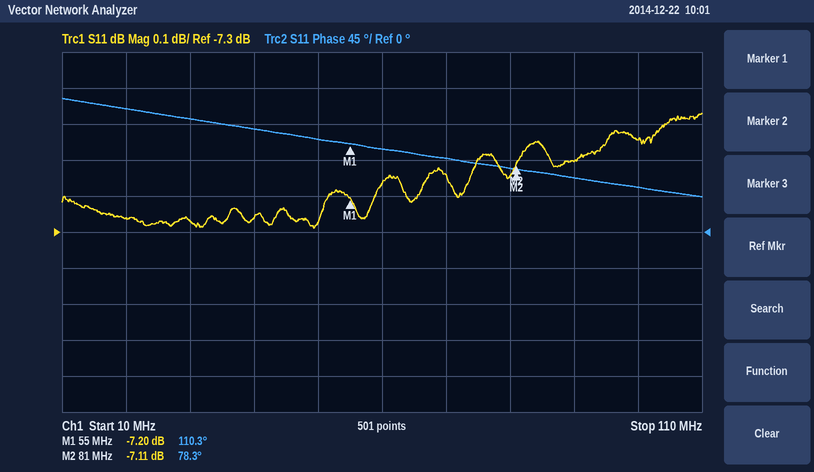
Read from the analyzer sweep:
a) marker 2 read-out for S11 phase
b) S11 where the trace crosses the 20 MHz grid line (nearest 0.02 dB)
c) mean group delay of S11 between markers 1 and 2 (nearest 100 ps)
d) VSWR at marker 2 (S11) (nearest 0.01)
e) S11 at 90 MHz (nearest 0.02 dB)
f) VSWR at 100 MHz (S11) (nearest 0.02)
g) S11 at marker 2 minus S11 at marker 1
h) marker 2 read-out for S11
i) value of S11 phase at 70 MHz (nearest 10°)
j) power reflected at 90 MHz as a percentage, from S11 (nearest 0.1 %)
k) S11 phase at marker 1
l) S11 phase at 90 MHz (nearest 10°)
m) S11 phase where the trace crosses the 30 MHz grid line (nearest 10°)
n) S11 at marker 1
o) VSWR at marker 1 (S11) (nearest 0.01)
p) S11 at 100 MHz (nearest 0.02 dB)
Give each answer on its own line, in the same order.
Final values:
78.3°
-7.26 dB
3.4 ns
2.58
-7.10 dB
2.60
0.09 dB
-7.11 dB
90°
19.5 %
110.3°
70°
140°
-7.20 dB
2.55
-7.04 dB
